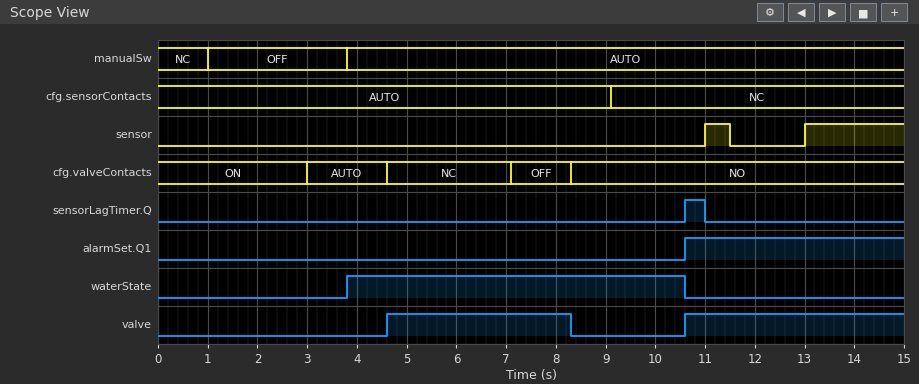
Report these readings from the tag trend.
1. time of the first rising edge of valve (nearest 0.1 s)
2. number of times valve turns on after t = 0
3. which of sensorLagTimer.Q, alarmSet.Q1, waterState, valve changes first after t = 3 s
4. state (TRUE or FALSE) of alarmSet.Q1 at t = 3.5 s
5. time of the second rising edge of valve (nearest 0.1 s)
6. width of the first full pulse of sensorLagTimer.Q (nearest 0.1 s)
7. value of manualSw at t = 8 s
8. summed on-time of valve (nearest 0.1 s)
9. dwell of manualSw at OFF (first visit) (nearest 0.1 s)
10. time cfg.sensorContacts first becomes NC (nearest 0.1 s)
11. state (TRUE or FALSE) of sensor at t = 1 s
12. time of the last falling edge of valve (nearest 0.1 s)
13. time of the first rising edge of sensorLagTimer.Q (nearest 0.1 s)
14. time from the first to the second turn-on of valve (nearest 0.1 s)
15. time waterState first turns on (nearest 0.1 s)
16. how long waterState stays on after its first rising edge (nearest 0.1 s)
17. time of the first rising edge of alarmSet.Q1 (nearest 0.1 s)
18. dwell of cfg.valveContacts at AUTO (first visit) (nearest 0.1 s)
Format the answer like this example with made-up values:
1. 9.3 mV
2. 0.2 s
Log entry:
1. 4.6 s
2. 2
3. waterState
4. FALSE
5. 10.6 s
6. 0.4 s
7. AUTO
8. 8.1 s
9. 2.8 s
10. 9.1 s
11. FALSE
12. 8.3 s
13. 10.6 s
14. 6.0 s
15. 3.8 s
16. 6.8 s
17. 10.6 s
18. 1.6 s
